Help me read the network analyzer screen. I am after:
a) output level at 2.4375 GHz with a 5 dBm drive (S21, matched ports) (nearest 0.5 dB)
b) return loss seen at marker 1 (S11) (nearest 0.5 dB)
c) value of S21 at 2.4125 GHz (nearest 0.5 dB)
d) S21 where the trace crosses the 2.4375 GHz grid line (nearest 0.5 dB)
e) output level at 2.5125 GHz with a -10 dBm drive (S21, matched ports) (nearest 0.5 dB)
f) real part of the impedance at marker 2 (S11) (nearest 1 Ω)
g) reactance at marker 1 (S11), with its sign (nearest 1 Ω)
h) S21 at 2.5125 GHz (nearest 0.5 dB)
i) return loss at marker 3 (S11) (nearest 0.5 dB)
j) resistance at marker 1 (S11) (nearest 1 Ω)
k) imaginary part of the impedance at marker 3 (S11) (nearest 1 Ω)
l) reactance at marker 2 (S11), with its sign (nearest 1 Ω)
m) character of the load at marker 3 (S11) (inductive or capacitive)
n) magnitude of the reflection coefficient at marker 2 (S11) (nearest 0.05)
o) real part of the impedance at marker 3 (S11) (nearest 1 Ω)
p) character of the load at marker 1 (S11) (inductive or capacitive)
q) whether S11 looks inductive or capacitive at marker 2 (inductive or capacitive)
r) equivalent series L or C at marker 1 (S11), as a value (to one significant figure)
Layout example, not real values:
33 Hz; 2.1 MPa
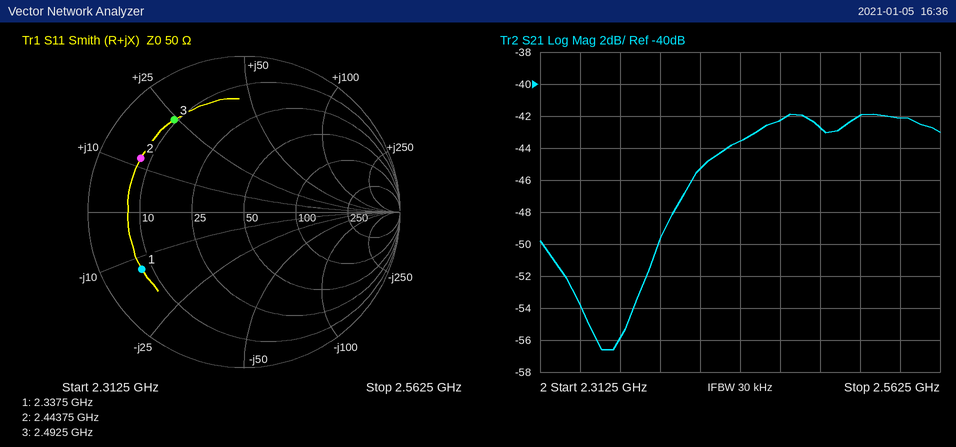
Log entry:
-38.5 dBm; 2.5 dB; -45.5 dB; -43.5 dB; -52.0 dBm; 8 Ω; -13 Ω; -42.0 dB; 2.5 dB; 8 Ω; +24 Ω; +12 Ω; inductive; 0.75; 9 Ω; capacitive; inductive; 5 pF
